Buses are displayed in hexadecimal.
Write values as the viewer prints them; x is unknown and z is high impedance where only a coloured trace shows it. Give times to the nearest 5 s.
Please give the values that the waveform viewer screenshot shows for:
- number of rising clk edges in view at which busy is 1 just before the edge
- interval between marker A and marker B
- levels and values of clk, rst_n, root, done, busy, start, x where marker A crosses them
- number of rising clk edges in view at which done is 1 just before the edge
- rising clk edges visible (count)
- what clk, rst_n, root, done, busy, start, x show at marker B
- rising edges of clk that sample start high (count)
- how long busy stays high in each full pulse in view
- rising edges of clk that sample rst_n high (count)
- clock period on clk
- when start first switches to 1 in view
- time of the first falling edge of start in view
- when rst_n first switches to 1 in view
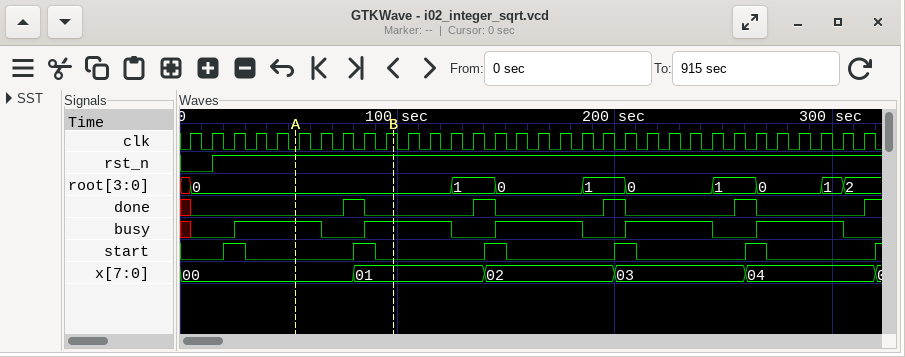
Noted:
20
45 s
clk=0, rst_n=1, root=0, done=0, busy=1, start=0, x=00
4
32
clk=1, rst_n=1, root=0, done=0, busy=1, start=0, x=01
5
40 s, 40 s, 40 s, 40 s, 40 s
30
10 s
20 s
30 s
15 s
